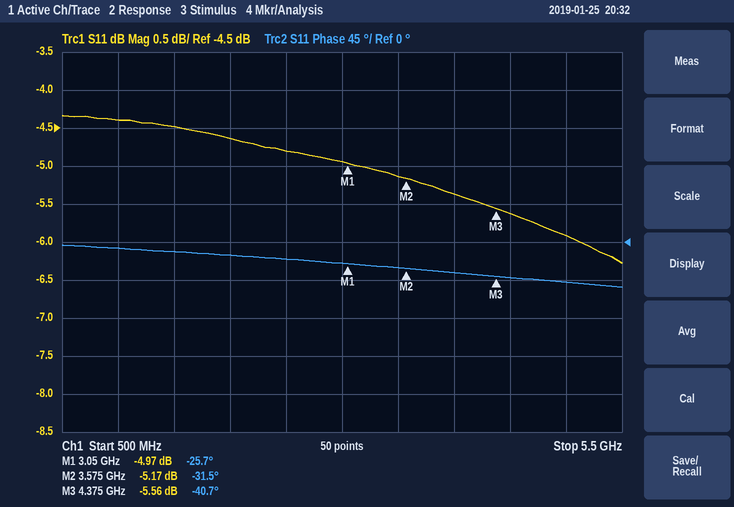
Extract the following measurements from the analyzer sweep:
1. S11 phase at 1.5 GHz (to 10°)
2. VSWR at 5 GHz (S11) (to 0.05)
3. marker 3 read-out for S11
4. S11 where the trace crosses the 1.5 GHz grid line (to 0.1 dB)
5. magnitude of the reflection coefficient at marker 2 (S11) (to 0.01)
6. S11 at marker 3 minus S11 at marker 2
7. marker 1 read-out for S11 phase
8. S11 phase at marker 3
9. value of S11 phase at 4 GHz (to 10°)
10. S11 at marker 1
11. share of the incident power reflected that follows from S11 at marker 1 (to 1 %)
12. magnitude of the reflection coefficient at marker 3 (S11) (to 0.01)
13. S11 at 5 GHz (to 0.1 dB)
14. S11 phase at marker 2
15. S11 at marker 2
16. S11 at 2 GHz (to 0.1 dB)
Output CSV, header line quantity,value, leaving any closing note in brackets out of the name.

quantity,value
S11 phase at 1.5 GHz,-10°
VSWR at 5 GHz (S11),3.05
marker 3 read-out for S11,-5.56 dB
S11 where the trace crosses the 1.5 GHz grid line,-4.5 dB
magnitude of the reflection coefficient at marker 2 (S11),0.55
S11 at marker 3 minus S11 at marker 2,-0.39 dB
marker 1 read-out for S11 phase,-25.7°
S11 phase at marker 3,-40.7°
value of S11 phase at 4 GHz,-40°
S11 at marker 1,-4.97 dB
share of the incident power reflected that follows from S11 at marker 1,32 %
magnitude of the reflection coefficient at marker 3 (S11),0.53
S11 at 5 GHz,-5.9 dB
S11 phase at marker 2,-31.5°
S11 at marker 2,-5.17 dB
S11 at 2 GHz,-4.6 dB
